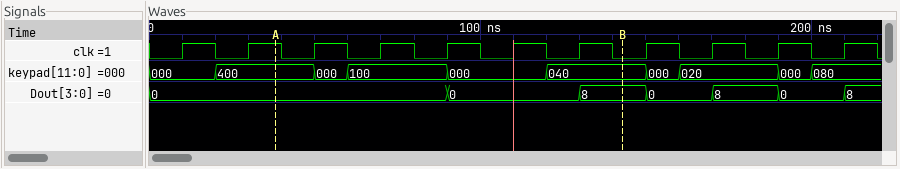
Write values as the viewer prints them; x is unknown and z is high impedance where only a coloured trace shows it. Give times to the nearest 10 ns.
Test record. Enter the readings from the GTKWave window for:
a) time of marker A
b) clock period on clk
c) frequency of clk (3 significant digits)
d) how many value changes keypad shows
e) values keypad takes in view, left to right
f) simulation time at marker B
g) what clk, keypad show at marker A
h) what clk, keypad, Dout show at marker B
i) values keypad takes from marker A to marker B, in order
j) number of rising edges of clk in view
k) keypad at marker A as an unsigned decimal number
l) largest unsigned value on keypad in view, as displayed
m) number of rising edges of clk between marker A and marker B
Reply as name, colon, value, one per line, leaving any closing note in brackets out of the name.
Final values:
time of marker A: 40 ns
clock period on clk: 20 ns
frequency of clk: 50.0 MHz
how many value changes keypad shows: 9
values keypad takes in view, left to right: 000, 400, 000, 100, 000, 040, 000, 020, 000, 080
simulation time at marker B: 140 ns
what clk, keypad show at marker A: clk=1, keypad=400
what clk, keypad, Dout show at marker B: clk=0, keypad=040, Dout=8
values keypad takes from marker A to marker B, in order: 400, 000, 100, 000, 040
number of rising edges of clk in view: 11
keypad at marker A as an unsigned decimal number: 1024
largest unsigned value on keypad in view, as displayed: 400
number of rising edges of clk between marker A and marker B: 5
